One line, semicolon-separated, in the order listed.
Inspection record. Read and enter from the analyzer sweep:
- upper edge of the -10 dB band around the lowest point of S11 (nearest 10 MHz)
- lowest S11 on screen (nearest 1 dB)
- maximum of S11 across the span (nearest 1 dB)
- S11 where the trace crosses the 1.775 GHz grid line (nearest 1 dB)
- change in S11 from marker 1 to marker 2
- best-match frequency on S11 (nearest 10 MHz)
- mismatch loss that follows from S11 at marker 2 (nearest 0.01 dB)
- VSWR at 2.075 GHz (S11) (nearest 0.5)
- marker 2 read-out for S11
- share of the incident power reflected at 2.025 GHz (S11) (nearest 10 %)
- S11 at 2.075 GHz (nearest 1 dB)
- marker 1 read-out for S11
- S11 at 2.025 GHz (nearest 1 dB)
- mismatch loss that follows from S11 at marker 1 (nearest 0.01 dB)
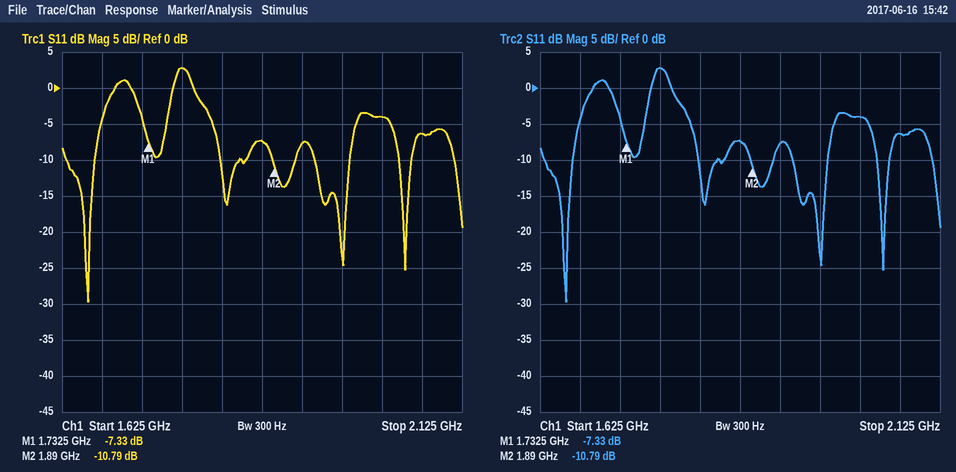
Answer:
1.67 GHz; -30 dB; 3 dB; 3 dB; -3.46 dB; 1.66 GHz; 0.38 dB; 3.0; -10.79 dB; 40 %; -6 dB; -7.33 dB; -4 dB; 0.89 dB
